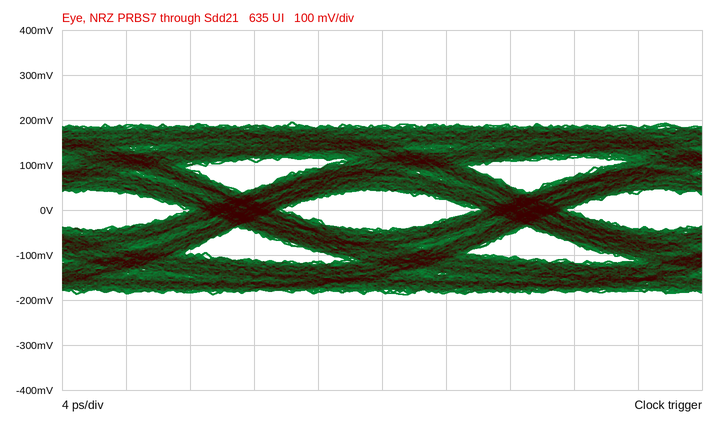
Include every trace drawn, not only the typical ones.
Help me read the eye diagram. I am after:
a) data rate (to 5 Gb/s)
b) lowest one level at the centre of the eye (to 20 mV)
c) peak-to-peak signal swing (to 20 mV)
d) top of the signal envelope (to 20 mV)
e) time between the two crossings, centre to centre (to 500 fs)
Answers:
55 Gb/s
40 mV
380 mV
200 mV
18.0 ps
